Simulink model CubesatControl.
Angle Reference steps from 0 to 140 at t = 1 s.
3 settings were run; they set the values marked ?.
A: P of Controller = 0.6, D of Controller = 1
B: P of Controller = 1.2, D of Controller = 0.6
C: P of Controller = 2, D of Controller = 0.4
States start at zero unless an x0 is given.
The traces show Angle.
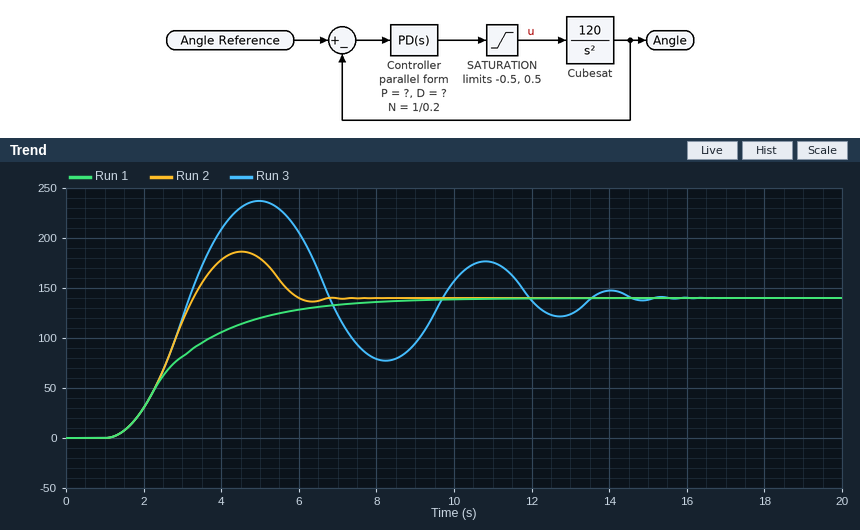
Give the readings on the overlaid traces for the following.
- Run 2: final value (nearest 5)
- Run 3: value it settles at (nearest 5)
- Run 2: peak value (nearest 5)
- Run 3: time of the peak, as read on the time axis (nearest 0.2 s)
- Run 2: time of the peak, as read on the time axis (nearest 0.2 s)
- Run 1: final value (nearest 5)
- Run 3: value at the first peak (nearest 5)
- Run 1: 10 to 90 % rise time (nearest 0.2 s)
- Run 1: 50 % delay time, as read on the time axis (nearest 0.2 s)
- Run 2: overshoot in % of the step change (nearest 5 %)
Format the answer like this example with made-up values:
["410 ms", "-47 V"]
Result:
["140", "140", "185", "5.0 s", "4.6 s", "140", "235", "4.0 s", "2.6 s", "35 %"]
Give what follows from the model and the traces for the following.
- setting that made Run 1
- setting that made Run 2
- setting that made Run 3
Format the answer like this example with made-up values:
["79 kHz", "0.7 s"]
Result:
["A", "B", "C"]
